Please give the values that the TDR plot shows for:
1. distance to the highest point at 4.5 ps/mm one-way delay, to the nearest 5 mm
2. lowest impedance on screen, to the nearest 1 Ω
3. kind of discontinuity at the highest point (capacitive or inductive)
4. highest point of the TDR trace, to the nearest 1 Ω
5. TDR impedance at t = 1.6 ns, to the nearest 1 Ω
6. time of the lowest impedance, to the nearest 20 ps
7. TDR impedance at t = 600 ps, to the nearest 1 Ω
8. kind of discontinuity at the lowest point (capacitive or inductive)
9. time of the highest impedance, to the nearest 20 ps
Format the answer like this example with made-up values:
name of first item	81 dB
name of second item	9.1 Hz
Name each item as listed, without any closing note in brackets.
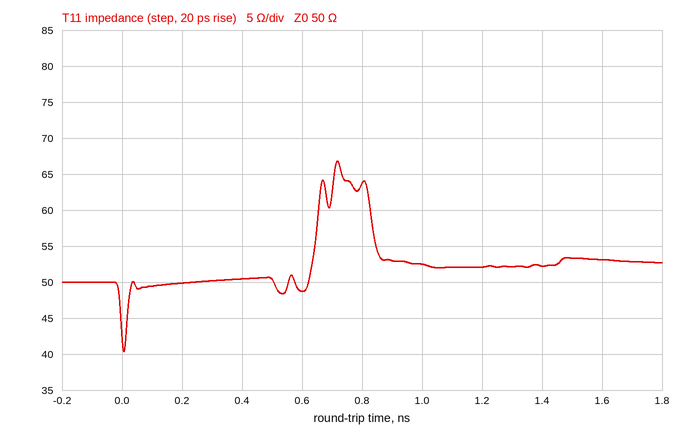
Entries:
distance to the highest point at 4.5 ps/mm one-way delay, to the nearest 5 mm	80 mm
lowest impedance on screen, to the nearest 1 Ω	40 Ω
kind of discontinuity at the highest point	inductive
highest point of the TDR trace, to the nearest 1 Ω	67 Ω
TDR impedance at t = 1.6 ns, to the nearest 1 Ω	53 Ω
time of the lowest impedance, to the nearest 20 ps	0 ps
TDR impedance at t = 600 ps, to the nearest 1 Ω	49 Ω
kind of discontinuity at the lowest point	capacitive
time of the highest impedance, to the nearest 20 ps	720 ps
